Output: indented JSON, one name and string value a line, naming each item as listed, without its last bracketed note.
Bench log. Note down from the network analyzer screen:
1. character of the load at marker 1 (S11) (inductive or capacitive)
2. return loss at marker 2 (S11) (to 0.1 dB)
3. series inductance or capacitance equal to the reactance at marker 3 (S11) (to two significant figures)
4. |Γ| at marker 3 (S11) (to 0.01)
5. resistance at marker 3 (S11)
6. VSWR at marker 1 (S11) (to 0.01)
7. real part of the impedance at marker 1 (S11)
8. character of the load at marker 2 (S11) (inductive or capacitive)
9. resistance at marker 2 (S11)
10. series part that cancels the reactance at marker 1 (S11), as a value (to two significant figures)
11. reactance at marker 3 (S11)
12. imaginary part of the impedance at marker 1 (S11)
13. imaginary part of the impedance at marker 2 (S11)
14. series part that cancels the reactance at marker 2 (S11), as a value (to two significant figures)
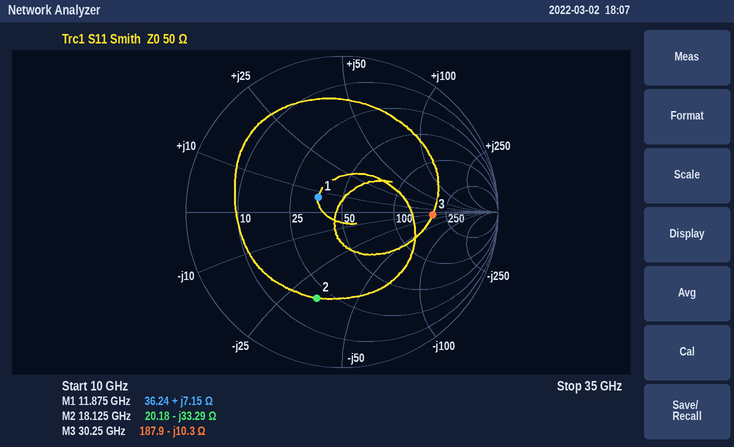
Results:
{
  "character of the load at marker 1 (S11)": "inductive",
  "return loss at marker 2 (S11)": "4.8 dB",
  "series inductance or capacitance equal to the reactance at marker 3 (S11)": "510 fF",
  "|Γ| at marker 3 (S11)": "0.58",
  "resistance at marker 3": "187.9 Ω",
  "VSWR at marker 1 (S11)": "1.44",
  "real part of the impedance at marker 1": "36.24 Ω",
  "character of the load at marker 2 (S11)": "capacitive",
  "resistance at marker 2": "20.18 Ω",
  "series part that cancels the reactance at marker 1 (S11), as a value": "1.9 pF",
  "reactance at marker 3": "-10.3 Ω",
  "imaginary part of the impedance at marker 1": "+7.15 Ω",
  "imaginary part of the impedance at marker 2": "-33.29 Ω",
  "series part that cancels the reactance at marker 2 (S11), as a value": "290 pH"
}
